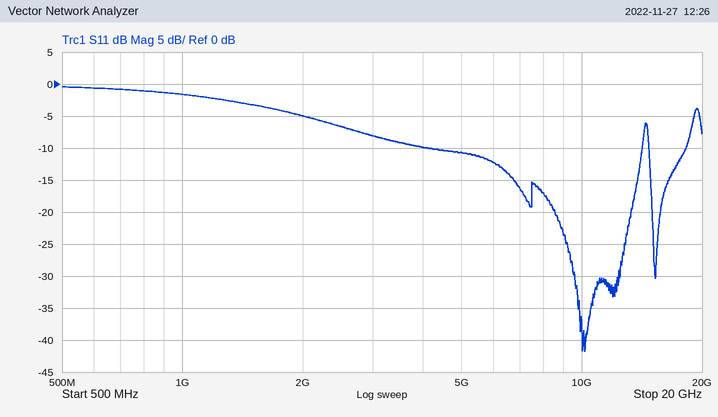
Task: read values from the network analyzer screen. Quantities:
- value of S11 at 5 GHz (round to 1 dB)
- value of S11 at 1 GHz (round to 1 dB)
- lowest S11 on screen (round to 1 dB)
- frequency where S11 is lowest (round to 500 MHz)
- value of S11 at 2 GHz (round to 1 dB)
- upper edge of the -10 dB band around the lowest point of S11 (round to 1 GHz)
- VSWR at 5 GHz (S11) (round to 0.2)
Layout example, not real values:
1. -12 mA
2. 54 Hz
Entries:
1. -11 dB
2. -2 dB
3. -42 dB
4. 10.0 GHz
5. -5 dB
6. 14 GHz
7. 1.8
